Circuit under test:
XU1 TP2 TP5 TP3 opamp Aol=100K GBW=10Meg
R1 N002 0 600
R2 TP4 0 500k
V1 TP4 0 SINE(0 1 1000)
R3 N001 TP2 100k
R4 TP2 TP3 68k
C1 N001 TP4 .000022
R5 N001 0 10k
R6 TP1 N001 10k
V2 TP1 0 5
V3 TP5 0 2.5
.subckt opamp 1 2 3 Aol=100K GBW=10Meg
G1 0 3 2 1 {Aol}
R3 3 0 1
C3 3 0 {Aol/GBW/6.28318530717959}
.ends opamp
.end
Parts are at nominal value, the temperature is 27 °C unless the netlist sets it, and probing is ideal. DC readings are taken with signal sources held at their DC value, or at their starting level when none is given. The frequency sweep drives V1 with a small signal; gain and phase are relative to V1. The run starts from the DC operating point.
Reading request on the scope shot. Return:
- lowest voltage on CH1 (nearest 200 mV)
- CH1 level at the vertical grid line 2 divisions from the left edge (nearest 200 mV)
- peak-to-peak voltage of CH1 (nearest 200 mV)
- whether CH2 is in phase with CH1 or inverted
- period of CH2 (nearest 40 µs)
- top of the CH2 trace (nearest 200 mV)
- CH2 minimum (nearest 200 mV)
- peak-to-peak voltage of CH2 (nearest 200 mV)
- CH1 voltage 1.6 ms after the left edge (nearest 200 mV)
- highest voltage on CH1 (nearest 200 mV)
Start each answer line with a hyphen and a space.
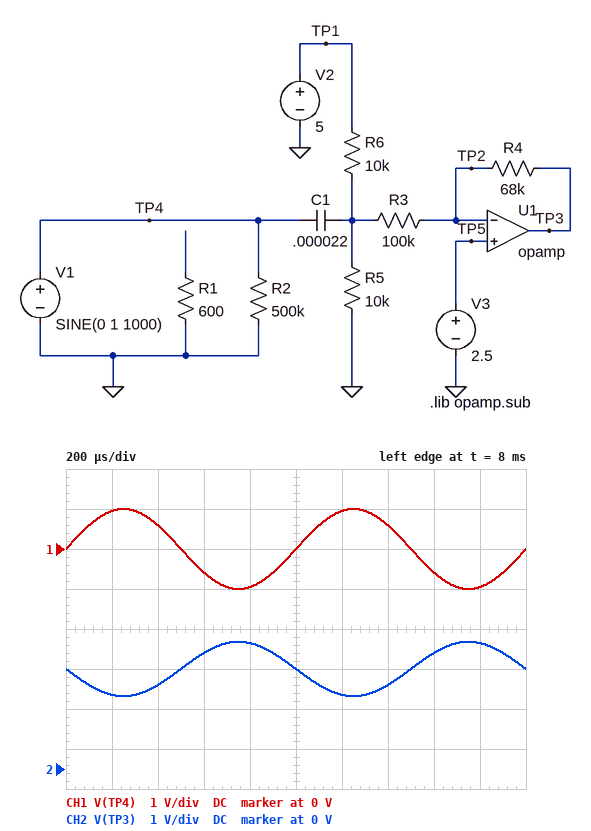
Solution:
- -1.0 V
- 600 mV
- 2.0 V
- inverted
- 1.00 ms
- 3.2 V
- 1.8 V
- 1.4 V
- -600 mV
- 1.0 V
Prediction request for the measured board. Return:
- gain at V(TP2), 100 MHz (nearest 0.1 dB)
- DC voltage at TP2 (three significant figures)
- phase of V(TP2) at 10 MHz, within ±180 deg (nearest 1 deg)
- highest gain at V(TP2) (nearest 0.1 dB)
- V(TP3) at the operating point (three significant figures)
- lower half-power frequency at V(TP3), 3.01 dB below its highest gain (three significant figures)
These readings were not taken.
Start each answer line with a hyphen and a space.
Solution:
- -7.9 dB
- 2.50 V
- 31 deg
- -7.9 dB
- 2.50 V
- 1.52 Hz
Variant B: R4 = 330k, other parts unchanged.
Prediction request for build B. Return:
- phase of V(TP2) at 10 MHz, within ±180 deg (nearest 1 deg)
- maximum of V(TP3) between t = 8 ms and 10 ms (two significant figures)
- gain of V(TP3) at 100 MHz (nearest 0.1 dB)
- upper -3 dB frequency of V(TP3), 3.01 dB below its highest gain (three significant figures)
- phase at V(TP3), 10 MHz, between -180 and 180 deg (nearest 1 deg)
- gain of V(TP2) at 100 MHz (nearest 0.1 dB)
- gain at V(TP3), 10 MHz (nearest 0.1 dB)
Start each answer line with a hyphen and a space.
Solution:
- 13 deg
- 5.8 V
- -22.3 dB
- 2.33 MHz
- 103 deg
- -2.3 dB
- -2.5 dB
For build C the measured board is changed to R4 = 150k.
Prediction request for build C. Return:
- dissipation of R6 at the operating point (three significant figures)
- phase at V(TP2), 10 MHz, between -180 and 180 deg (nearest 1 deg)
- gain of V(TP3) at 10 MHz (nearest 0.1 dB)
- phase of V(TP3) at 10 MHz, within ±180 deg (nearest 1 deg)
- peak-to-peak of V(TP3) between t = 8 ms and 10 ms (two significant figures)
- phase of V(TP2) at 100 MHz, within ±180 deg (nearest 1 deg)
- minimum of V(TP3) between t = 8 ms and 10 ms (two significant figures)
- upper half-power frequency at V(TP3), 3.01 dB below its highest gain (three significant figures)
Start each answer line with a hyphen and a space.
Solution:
- 625 µW
- 22 deg
- -5.1 dB
- 112 deg
- 3.0 V
- 2 deg
- 1.0 V
- 4.00 MHz
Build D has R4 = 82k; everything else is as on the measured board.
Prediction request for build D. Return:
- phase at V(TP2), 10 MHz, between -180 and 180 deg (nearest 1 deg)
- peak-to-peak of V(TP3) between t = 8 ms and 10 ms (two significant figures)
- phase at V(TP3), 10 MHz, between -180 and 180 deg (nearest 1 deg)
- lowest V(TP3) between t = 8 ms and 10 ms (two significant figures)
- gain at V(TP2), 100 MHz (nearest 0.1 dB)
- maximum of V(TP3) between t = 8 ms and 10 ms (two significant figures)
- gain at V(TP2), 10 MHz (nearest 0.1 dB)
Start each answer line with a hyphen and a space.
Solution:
- 29 deg
- 1.6 V
- 119 deg
- 1.7 V
- -6.9 dB
- 3.3 V
- -8.1 dB
